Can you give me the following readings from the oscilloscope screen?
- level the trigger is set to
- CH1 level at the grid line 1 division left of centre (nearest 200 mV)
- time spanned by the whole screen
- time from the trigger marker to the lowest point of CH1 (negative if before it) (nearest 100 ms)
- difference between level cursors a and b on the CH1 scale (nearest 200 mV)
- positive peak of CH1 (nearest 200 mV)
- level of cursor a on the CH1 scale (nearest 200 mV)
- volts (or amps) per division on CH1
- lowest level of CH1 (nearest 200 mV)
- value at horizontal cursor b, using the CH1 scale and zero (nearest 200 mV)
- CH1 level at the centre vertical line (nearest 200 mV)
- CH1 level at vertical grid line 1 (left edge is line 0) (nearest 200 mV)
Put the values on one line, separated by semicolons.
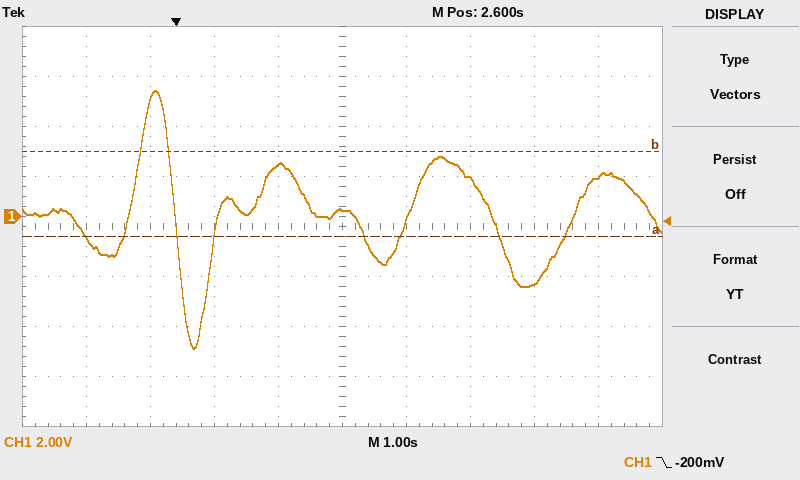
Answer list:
-200 mV; 2.0 V; 10 s; +300 ms; 3.4 V; 5.0 V; -800 mV; 2 V; -5.2 V; 2.6 V; 200 mV; -800 mV
